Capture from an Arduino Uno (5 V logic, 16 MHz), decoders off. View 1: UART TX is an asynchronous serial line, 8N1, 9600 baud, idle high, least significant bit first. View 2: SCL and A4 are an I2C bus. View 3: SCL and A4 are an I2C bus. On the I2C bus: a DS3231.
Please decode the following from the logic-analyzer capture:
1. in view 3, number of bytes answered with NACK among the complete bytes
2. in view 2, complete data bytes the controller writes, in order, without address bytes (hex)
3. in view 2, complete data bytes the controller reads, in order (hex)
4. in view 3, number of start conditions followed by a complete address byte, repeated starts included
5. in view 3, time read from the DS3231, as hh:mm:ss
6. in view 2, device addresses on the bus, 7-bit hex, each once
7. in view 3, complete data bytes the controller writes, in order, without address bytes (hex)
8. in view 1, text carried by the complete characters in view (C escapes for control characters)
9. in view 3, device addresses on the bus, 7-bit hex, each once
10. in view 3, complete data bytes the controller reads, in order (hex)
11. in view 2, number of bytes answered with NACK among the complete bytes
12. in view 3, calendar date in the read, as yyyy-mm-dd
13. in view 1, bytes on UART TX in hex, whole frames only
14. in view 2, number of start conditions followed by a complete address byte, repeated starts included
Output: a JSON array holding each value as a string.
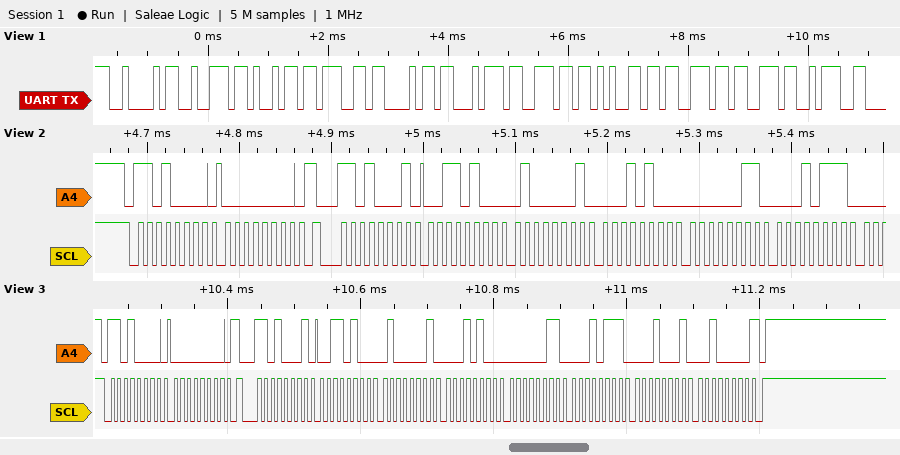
["1", "00", "34 41 14 03 17", "2", "14:41:34", "0x68", "00", "\"Brightness:\"", "0x68", "34 41 14 03 17 11 20", "0", "2020-11-17", "0x42 0x72 0x69 0x67 0x68 0x74 0x6E 0x65 0x73 0x73 0x3A", "2"]
